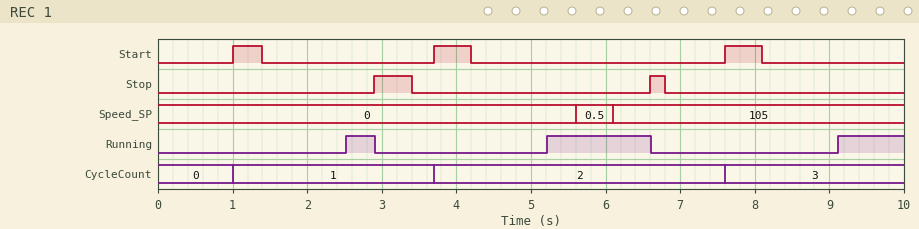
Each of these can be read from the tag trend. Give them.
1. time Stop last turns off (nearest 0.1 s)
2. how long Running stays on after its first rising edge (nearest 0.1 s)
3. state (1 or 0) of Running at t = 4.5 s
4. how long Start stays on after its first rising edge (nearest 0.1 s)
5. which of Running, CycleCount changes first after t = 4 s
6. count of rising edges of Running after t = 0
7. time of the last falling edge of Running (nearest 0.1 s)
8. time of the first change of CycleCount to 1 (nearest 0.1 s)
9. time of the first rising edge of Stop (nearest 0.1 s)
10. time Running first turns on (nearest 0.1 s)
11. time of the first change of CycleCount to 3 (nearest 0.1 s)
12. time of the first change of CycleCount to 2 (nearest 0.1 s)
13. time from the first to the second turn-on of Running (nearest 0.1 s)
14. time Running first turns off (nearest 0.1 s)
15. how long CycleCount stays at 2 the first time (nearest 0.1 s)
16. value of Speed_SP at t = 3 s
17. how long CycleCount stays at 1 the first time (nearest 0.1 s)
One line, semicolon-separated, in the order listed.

6.8 s; 0.4 s; 0; 0.4 s; Running; 3; 6.6 s; 1.0 s; 2.9 s; 2.5 s; 7.6 s; 3.7 s; 2.7 s; 2.9 s; 3.9 s; 0; 2.7 s
